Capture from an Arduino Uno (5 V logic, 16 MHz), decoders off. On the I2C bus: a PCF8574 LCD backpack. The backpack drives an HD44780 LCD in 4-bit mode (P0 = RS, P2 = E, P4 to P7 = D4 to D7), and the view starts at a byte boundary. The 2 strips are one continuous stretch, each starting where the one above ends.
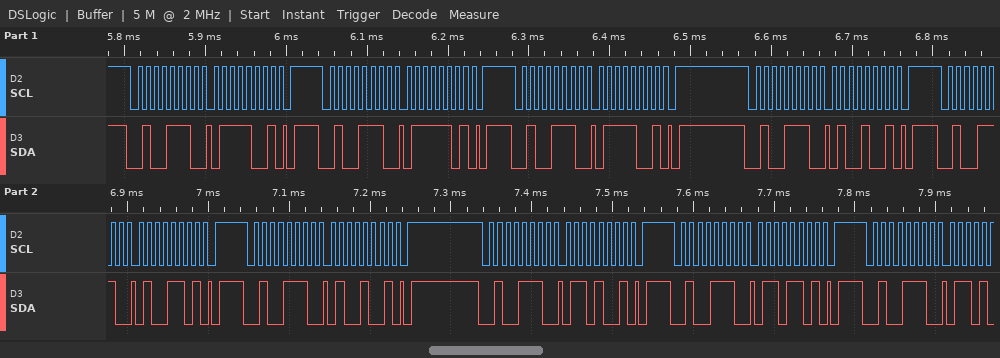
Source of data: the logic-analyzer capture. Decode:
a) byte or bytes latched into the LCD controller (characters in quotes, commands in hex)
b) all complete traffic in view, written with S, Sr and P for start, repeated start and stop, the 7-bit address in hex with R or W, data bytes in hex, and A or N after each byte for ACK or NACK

't'
S 27W A 79 A P S 27W A 7D A P S 27W A 79 A P S 27W A 49 A P S 27W A 4D A P S 27W A 49 A P S 27W A 69 A P S 27W A 6D A P S 27W A
